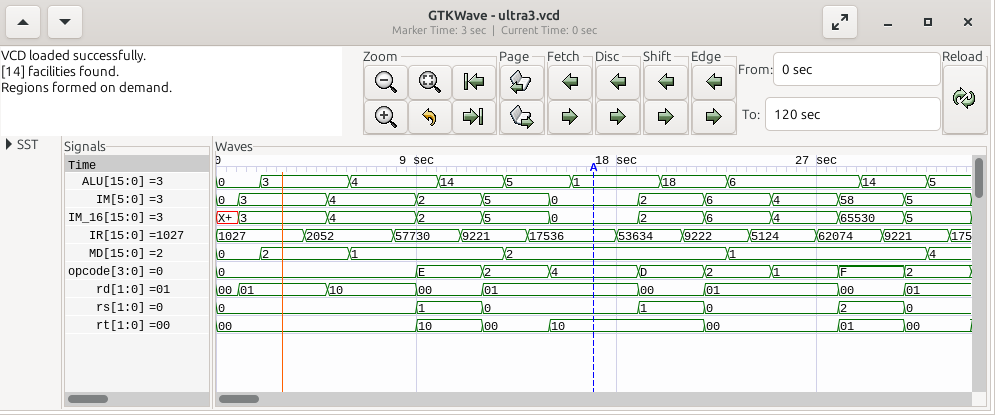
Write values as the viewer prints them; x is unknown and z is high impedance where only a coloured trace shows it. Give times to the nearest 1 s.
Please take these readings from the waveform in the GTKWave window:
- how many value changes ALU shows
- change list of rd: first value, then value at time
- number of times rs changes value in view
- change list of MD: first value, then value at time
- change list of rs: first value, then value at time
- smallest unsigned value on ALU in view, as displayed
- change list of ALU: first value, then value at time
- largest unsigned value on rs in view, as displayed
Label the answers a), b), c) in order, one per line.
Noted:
a) 9
b) 00, 01 at 1 s, 10 at 5 s, 00 at 9 s, 01 at 12 s, 00 at 19 s, 01 at 22 s, 00 at 28 s, 01 at 31 s
c) 6
d) 0, 2 at 2 s, 1 at 6 s, 2 at 13 s, 1 at 23 s, 4 at 32 s
e) 0, 1 at 9 s, 0 at 12 s, 1 at 19 s, 0 at 22 s, 2 at 28 s, 0 at 31 s
f) 0
g) 0, 3 at 2 s, 4 at 6 s, 14 at 10 s, 5 at 13 s, 1 at 16 s, 18 at 20 s, 6 at 23 s, 14 at 29 s, 5 at 32 s
h) 2
